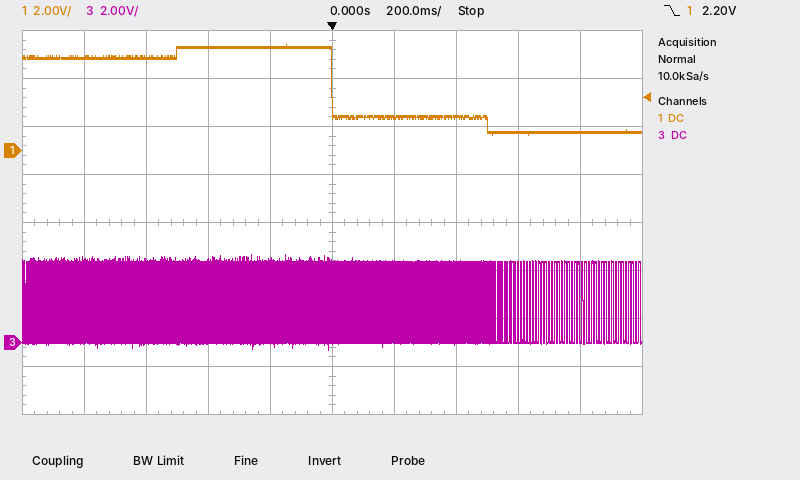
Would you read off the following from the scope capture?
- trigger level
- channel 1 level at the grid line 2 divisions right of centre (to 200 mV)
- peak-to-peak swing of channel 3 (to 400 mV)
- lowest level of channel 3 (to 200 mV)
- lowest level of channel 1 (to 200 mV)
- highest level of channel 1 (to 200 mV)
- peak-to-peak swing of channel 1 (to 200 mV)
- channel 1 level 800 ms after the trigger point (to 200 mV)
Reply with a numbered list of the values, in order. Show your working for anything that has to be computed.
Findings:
1. 2.20 V
2. 1.4 V
3. 4.0 V
4. -400 mV
5. 600 mV
6. 4.4 V
7. 4.4 V − (600 mV) = 3.8 V
8. 800 mV
